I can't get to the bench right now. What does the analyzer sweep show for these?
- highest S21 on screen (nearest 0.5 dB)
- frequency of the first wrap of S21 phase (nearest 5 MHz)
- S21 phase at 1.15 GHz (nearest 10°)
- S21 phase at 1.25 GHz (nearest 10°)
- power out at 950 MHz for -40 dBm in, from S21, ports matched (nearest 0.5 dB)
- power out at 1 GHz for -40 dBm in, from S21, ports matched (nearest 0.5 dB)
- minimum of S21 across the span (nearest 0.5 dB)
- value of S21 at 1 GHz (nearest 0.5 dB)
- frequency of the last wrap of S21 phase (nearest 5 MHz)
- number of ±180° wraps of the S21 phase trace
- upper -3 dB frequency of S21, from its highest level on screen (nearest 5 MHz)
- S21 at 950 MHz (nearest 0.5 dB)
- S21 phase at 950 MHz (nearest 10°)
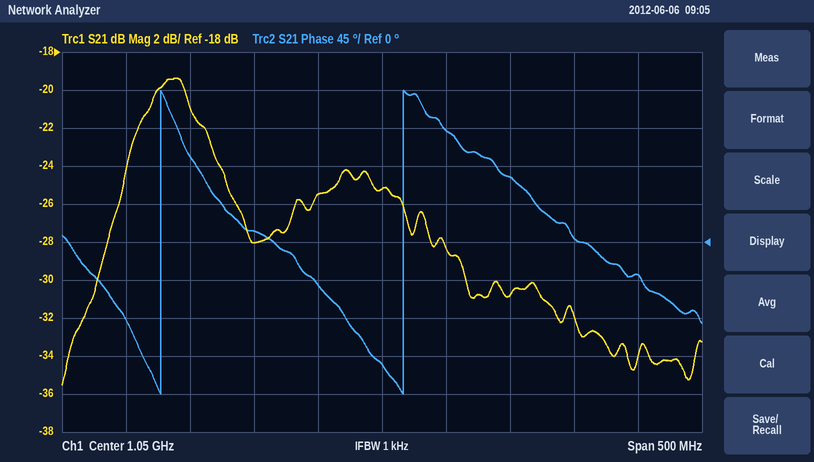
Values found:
-19.5 dB
875 MHz
80°
-40°
-68.0 dBm
-65.5 dBm
-35.5 dB
-25.5 dB
1.065 GHz
2
915 MHz
-28.0 dB
10°
